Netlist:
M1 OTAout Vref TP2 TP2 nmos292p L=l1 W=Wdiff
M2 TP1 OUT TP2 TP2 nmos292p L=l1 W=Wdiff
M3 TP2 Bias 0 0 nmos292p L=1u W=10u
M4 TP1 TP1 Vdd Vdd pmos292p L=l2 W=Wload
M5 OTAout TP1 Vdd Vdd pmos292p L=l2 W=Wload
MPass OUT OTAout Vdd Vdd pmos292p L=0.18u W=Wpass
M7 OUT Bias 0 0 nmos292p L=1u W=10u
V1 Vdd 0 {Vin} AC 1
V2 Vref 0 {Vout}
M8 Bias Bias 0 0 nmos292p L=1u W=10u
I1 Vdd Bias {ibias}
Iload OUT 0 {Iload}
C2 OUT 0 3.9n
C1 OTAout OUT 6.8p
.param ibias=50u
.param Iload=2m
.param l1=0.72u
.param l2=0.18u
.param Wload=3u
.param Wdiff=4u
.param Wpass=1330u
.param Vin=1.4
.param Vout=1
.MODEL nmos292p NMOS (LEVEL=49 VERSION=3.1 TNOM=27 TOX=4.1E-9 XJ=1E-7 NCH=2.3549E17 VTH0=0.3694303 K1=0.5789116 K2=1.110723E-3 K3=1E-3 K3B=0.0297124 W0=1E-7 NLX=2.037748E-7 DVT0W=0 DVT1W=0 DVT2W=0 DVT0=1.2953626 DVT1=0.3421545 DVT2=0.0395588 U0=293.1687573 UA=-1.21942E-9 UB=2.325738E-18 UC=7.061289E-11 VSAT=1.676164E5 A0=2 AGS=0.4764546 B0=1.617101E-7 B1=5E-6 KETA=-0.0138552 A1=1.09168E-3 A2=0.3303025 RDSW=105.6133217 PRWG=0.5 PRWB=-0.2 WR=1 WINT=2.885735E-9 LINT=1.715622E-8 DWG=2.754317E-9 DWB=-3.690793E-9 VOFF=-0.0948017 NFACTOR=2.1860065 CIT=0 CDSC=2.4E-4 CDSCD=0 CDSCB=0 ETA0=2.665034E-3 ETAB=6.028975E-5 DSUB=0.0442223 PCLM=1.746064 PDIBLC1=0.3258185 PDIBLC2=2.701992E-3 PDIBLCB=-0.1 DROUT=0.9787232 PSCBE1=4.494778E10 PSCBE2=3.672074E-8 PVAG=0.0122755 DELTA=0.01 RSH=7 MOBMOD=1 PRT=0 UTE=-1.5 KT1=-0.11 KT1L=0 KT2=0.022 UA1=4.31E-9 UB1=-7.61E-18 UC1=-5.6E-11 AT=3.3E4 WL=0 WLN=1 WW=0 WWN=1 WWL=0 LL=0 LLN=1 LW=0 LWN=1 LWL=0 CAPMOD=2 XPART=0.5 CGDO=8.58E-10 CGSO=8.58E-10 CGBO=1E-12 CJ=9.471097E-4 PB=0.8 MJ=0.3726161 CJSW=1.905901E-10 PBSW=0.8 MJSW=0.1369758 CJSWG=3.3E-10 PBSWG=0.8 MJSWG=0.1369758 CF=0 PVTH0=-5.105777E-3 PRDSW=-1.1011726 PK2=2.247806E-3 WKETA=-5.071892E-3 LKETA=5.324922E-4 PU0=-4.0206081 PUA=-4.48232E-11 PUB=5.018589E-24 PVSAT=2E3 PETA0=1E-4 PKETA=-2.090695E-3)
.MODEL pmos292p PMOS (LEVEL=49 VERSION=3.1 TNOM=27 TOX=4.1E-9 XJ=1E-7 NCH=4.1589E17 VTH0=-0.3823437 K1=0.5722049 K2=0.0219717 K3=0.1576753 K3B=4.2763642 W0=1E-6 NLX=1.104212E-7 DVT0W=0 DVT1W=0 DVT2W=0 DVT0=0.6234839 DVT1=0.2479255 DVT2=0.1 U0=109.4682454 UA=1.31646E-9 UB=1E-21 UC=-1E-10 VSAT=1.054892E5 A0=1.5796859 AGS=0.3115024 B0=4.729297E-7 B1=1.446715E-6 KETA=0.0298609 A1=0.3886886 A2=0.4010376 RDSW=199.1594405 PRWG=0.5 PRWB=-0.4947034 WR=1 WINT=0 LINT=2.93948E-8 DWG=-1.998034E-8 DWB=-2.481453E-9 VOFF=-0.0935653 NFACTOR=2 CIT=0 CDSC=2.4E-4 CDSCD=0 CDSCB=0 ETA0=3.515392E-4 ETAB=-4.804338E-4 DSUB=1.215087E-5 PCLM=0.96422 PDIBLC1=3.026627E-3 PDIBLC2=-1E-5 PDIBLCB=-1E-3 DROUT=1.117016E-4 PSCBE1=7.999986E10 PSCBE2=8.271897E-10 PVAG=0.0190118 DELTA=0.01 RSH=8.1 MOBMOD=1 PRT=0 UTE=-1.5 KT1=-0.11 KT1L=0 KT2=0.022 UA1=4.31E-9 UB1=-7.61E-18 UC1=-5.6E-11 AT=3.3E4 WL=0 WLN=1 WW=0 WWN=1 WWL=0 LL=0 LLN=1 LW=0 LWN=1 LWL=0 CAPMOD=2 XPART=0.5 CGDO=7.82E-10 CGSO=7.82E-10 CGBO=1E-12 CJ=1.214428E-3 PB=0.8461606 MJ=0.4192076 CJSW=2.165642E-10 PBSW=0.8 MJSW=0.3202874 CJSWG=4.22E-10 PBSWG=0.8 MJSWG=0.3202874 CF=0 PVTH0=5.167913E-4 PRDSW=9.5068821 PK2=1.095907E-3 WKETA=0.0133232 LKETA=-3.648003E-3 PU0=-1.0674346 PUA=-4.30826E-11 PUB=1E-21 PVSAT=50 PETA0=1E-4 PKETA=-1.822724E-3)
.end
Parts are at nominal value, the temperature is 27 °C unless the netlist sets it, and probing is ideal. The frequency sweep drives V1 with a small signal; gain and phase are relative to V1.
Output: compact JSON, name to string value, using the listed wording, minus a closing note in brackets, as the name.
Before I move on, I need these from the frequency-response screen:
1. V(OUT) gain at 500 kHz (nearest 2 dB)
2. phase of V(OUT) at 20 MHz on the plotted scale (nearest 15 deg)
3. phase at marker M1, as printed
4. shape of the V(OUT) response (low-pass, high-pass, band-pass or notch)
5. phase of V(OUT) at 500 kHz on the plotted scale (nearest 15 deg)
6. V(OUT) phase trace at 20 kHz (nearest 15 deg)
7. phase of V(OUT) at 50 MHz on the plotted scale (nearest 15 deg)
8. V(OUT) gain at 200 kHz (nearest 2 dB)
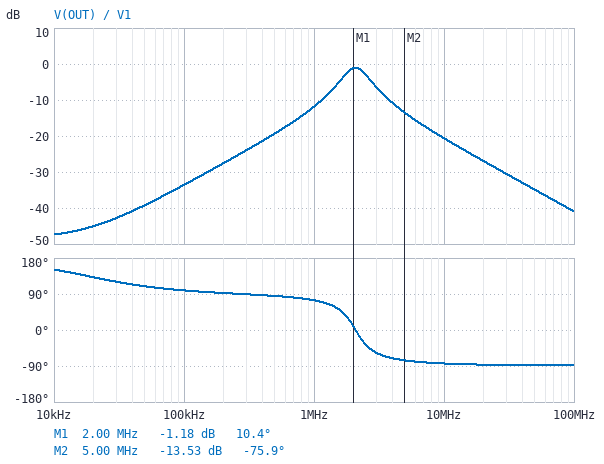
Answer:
{"V(OUT) gain at 500 kHz": "-20 dB", "phase of V(OUT) at 20 MHz on the plotted scale": "-90 deg", "phase at marker M1, as printed": "10.4 deg", "shape of the V(OUT) response": "band-pass", "phase of V(OUT) at 500 kHz on the plotted scale": "90 deg", "V(OUT) phase trace at 20 kHz": "135 deg", "phase of V(OUT) at 50 MHz on the plotted scale": "-90 deg", "V(OUT) gain at 200 kHz": "-28 dB"}
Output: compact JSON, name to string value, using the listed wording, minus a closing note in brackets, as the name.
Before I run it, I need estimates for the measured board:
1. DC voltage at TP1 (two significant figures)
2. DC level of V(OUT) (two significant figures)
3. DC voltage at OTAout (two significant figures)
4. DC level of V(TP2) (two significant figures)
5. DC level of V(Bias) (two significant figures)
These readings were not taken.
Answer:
{"DC voltage at TP1": "750 mV", "DC level of V(OUT)": "1.0 V", "DC voltage at OTAout": "840 mV", "DC level of V(TP2)": "380 mV", "DC level of V(Bias)": "620 mV"}
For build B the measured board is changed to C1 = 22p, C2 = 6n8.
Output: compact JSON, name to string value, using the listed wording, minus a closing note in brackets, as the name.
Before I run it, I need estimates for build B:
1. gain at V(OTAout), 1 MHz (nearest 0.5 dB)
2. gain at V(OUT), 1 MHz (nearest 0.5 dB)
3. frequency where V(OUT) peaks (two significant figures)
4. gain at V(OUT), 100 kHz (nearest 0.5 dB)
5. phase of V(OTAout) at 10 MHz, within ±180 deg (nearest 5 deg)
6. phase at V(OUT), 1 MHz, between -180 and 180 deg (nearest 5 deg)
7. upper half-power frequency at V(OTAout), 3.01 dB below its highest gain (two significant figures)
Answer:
{"gain at V(OTAout), 1 MHz": "5.0 dB", "gain at V(OUT), 1 MHz": "-0.5 dB", "frequency where V(OUT) peaks": "990 kHz", "gain at V(OUT), 100 kHz": "-24.5 dB", "phase of V(OTAout) at 10 MHz, within ±180 deg": "-40 deg", "phase at V(OUT), 1 MHz, between -180 and 180 deg": "0 deg", "upper half-power frequency at V(OTAout), 3.01 dB below its highest gain": "1.2 MHz"}
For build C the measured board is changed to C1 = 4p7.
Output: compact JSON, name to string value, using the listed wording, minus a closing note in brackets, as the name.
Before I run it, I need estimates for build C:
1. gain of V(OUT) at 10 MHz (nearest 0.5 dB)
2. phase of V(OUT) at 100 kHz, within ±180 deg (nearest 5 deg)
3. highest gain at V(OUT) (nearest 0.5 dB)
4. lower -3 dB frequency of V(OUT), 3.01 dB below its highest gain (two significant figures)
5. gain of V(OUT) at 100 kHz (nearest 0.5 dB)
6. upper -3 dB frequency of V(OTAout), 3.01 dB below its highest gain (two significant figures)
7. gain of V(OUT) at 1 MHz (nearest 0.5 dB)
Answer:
{"gain of V(OUT) at 10 MHz": "-21.0 dB", "phase of V(OUT) at 100 kHz, within ±180 deg": "105 deg", "highest gain at V(OUT)": "-1.5 dB", "lower -3 dB frequency of V(OUT), 3.01 dB below its highest gain": "1.9 MHz", "gain of V(OUT) at 100 kHz": "-36.0 dB", "upper -3 dB frequency of V(OTAout), 3.01 dB below its highest gain": "2.7 MHz", "gain of V(OUT) at 1 MHz": "-15.0 dB"}
